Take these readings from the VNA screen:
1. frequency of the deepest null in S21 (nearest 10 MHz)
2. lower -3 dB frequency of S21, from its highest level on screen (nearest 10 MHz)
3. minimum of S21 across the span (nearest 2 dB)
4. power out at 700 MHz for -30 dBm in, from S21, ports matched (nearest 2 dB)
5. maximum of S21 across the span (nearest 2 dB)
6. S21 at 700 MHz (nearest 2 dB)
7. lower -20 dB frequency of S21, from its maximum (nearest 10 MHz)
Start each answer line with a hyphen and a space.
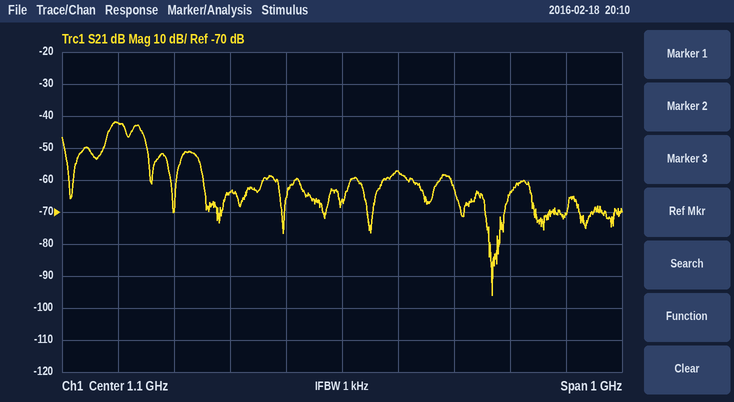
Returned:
- 1.37 GHz
- 680 MHz
- -96 dB
- -72 dBm
- -42 dB
- -42 dB
- 620 MHz
